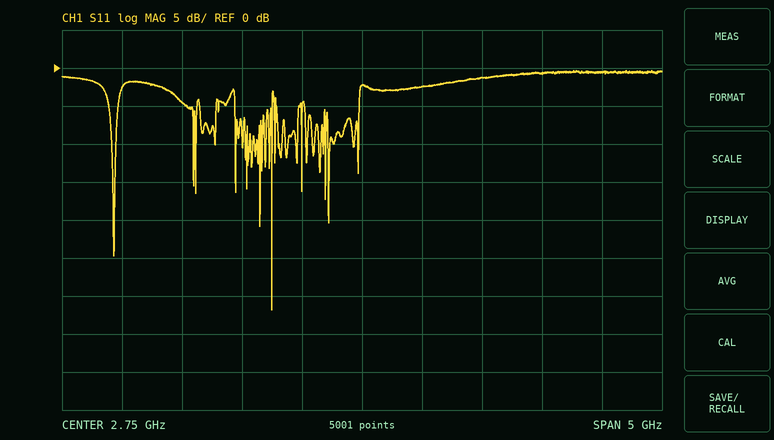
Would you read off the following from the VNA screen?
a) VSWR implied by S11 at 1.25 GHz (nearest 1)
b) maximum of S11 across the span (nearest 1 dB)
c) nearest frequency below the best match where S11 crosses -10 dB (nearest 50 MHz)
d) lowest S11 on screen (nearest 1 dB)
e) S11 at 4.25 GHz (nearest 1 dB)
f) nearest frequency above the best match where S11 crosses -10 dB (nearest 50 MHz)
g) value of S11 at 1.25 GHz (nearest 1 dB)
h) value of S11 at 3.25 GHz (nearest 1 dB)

4
0 dB
2.00 GHz
-32 dB
-1 dB
2.00 GHz
-5 dB
-2 dB
